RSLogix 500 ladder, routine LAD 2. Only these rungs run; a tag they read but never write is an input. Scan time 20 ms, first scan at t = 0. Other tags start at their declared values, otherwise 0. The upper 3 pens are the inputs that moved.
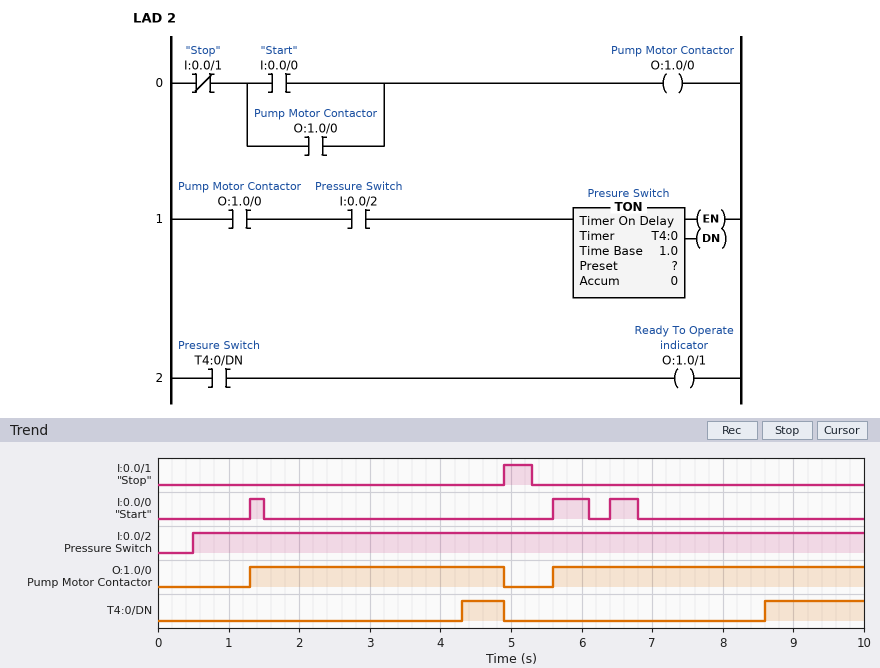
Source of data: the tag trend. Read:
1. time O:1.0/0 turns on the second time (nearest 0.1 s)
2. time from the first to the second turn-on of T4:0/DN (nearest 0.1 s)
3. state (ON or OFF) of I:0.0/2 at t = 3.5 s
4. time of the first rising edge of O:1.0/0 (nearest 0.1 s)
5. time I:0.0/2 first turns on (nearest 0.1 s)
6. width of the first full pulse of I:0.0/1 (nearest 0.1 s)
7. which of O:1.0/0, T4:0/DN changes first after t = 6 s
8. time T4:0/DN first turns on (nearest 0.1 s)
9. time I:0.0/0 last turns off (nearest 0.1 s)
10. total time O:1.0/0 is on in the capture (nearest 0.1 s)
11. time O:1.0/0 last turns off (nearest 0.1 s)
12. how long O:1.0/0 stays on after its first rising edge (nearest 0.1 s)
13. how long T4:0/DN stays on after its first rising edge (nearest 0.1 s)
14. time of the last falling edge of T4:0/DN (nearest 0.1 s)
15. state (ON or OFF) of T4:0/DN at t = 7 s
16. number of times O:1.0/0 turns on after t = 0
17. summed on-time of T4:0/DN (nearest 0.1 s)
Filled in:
5.6 s
4.3 s
ON
1.3 s
0.5 s
0.4 s
T4:0/DN
4.3 s
6.8 s
8.0 s
4.9 s
3.6 s
0.6 s
4.9 s
OFF
2
2.0 s
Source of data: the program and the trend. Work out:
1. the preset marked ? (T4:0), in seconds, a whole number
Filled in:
3 s
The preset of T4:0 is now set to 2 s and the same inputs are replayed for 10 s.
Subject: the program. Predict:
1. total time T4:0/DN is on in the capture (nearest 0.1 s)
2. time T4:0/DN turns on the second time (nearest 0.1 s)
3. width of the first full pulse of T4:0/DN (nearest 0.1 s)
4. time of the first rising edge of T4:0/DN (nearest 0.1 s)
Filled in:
4.0 s
7.6 s
1.6 s
3.3 s
